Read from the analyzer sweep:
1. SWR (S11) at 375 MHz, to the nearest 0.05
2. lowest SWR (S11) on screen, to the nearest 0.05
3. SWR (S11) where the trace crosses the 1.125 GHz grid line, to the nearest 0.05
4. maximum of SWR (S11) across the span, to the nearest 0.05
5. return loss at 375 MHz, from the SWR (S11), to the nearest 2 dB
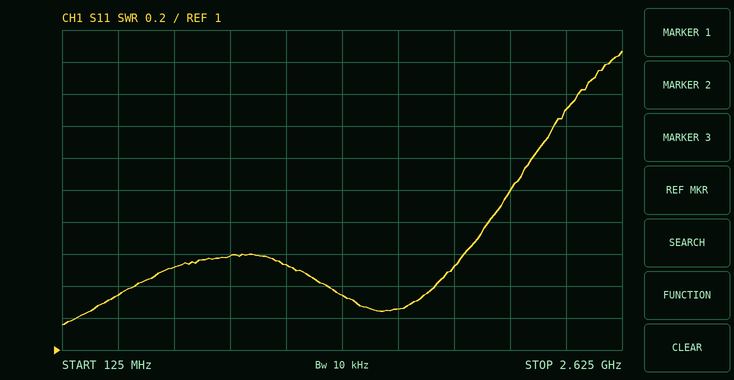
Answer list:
1.35
1.15
1.55
2.85
16 dB
